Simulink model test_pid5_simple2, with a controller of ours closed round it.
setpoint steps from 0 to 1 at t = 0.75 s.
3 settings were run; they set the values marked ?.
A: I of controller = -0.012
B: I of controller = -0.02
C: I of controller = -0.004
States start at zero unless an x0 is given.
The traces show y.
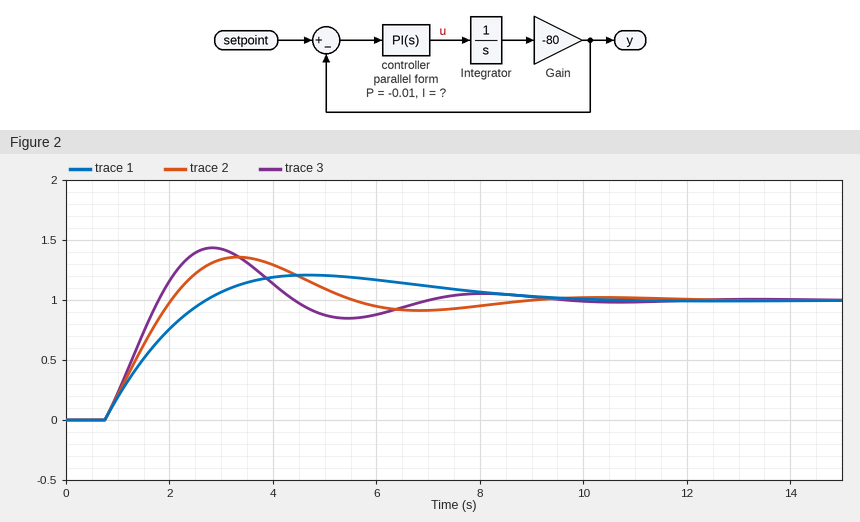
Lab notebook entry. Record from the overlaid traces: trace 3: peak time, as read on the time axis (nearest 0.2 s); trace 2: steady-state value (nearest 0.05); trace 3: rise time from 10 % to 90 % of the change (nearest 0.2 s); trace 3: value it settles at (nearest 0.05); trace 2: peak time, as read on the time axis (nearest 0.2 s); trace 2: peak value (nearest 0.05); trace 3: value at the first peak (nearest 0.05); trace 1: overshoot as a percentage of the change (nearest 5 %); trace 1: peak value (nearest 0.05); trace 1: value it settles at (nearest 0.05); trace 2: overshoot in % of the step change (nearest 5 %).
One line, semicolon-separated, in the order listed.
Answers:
2.8 s; 1.00; 0.8 s; 1.00; 3.4 s; 1.35; 1.45; 20 %; 1.20; 1.00; 35 %
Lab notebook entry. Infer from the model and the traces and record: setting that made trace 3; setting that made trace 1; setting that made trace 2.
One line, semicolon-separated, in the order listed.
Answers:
B; C; A
